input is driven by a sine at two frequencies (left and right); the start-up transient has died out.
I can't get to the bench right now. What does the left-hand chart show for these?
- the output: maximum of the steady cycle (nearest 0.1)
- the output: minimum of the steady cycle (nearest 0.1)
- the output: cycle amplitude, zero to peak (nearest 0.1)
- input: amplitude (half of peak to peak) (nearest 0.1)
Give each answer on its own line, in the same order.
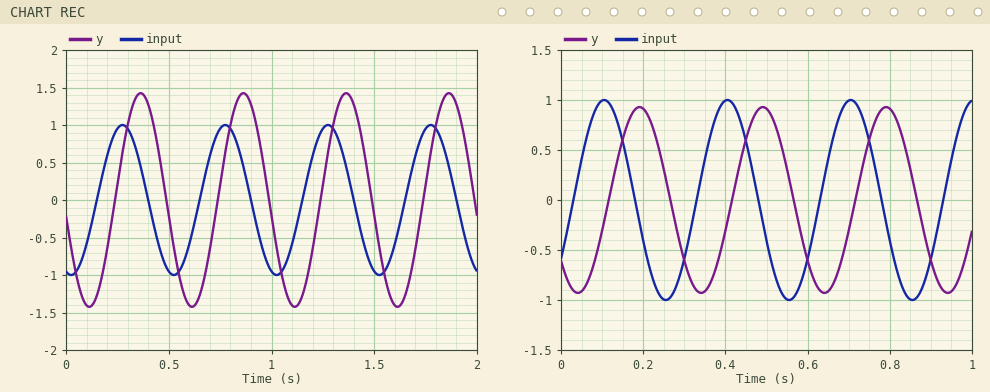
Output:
1.4
-1.4
1.4
1.0
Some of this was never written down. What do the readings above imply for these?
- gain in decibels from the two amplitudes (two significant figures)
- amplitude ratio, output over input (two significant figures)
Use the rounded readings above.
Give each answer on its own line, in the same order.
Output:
2.9 dB
1.4
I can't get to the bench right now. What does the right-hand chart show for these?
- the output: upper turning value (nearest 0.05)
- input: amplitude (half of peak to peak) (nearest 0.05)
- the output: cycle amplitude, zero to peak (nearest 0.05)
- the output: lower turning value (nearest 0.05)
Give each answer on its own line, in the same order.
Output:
0.95
1.00
0.95
-0.95
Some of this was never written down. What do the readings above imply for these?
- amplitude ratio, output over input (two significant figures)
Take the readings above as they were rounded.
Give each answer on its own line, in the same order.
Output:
0.95
